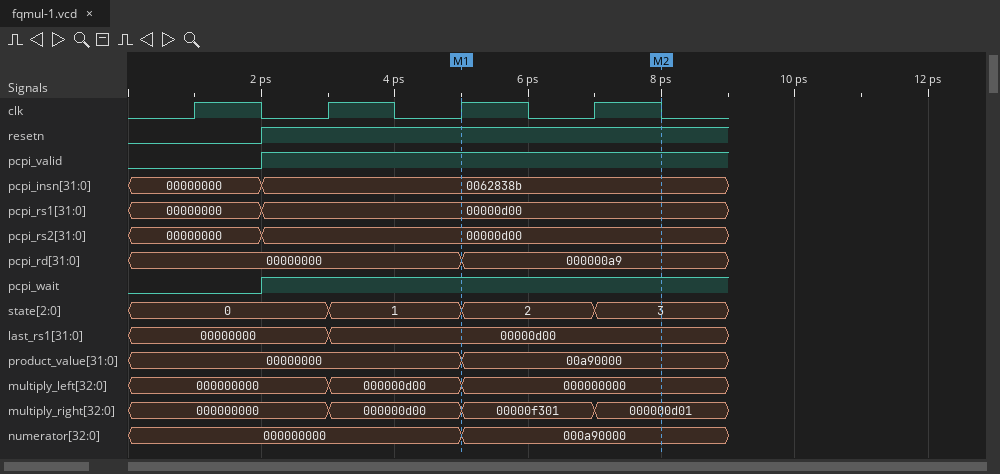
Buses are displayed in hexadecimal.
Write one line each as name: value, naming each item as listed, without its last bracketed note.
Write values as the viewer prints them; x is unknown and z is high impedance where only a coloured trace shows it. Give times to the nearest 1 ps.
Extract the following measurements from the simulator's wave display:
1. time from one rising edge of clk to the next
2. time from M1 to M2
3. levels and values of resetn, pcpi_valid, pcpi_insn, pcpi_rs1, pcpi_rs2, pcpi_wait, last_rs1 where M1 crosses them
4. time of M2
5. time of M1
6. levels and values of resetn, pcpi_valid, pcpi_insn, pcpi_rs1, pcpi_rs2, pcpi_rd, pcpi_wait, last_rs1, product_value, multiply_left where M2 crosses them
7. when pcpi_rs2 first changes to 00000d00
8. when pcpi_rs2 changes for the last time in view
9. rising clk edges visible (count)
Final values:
time from one rising edge of clk to the next: 2 ps
time from M1 to M2: 3 ps
levels and values of resetn, pcpi_valid, pcpi_insn, pcpi_rs1, pcpi_rs2, pcpi_wait, last_rs1 where M1 crosses them: resetn=1, pcpi_valid=1, pcpi_insn=0062838b, pcpi_rs1=00000d00, pcpi_rs2=00000d00, pcpi_wait=1, last_rs1=00000d00
time of M2: 8 ps
time of M1: 5 ps
levels and values of resetn, pcpi_valid, pcpi_insn, pcpi_rs1, pcpi_rs2, pcpi_rd, pcpi_wait, last_rs1, product_value, multiply_left where M2 crosses them: resetn=1, pcpi_valid=1, pcpi_insn=0062838b, pcpi_rs1=00000d00, pcpi_rs2=00000d00, pcpi_rd=000000a9, pcpi_wait=1, last_rs1=00000d00, product_value=00a90000, multiply_left=000000000
when pcpi_rs2 first changes to 00000d00: 2 ps
when pcpi_rs2 changes for the last time in view: 2 ps
rising clk edges visible: 4
